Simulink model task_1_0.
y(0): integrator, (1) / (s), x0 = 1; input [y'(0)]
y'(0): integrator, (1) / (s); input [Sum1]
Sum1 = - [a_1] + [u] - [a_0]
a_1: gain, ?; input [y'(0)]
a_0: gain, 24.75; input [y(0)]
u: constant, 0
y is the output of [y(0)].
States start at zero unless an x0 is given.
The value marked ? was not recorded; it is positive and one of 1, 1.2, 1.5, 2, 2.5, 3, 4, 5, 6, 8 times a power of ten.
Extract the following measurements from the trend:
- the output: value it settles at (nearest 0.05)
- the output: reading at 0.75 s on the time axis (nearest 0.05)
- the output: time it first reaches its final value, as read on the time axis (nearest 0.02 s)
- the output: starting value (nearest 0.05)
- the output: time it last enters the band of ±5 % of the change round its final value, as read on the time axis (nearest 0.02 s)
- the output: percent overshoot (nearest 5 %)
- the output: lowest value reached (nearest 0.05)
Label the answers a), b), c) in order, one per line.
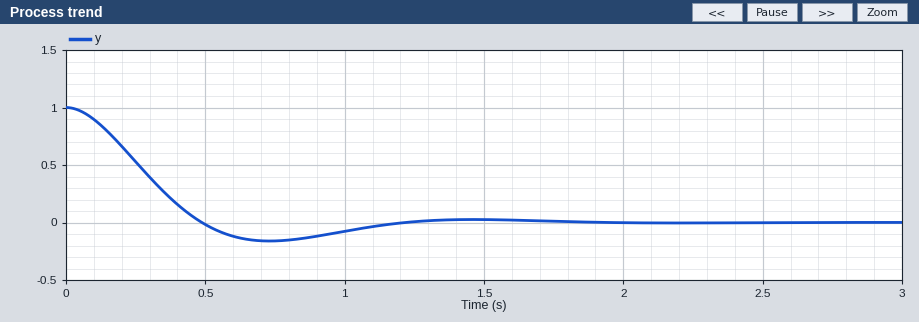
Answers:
a) 0.00
b) -0.15
c) 0.48 s
d) 1.00
e) 1.06 s
f) 15 %
g) -0.15
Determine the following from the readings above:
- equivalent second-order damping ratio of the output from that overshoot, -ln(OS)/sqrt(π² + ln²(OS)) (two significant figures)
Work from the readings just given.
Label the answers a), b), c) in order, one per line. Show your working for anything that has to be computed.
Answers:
a) ln(0.15) = -1.897; 1.897 / sqrt(9.870 + 3.599) = 0.52
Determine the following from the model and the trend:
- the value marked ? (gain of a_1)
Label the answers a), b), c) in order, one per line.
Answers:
a) 5
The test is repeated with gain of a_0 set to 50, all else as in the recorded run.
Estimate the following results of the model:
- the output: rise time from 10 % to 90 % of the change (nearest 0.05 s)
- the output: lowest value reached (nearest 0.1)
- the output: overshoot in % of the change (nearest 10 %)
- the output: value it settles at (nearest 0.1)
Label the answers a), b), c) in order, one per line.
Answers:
a) 0.20 s
b) -0.3
c) 30 %
d) 0.0
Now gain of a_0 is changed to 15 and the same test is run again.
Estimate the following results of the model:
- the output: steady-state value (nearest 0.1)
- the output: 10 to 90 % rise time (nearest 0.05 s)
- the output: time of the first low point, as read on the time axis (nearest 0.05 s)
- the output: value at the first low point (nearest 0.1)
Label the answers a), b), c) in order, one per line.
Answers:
a) 0.0
b) 0.50 s
c) 1.05 s
d) -0.1
